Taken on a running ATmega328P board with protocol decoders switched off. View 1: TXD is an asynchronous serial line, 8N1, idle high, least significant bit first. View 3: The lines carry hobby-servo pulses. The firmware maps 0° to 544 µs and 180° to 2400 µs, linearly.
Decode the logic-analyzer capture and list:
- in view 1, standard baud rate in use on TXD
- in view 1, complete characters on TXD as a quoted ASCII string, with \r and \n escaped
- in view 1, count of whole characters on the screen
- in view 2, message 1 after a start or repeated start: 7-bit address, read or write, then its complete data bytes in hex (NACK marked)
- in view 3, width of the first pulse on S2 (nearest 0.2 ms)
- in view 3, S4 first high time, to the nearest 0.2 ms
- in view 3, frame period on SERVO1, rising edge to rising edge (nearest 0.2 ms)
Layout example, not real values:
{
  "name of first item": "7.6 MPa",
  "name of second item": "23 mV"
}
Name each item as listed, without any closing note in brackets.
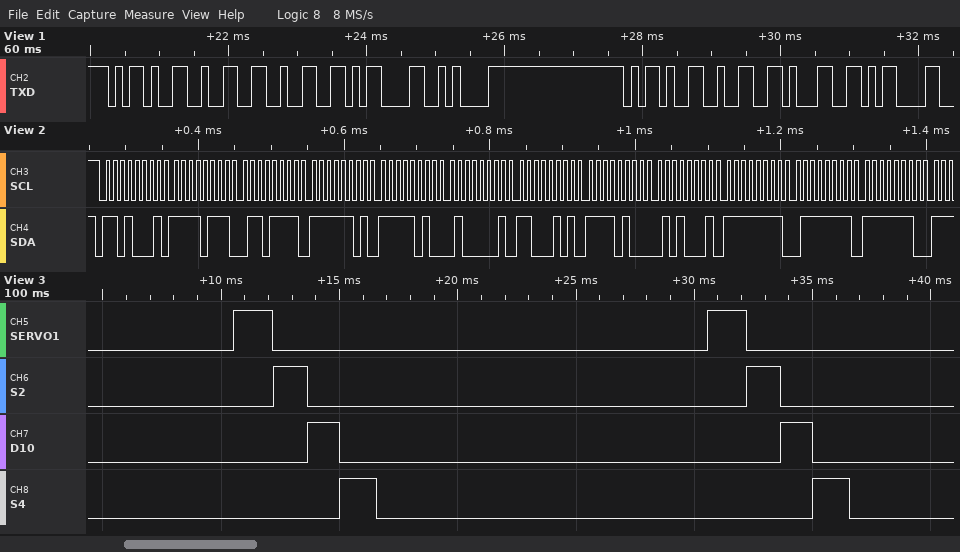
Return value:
{
  "in view 1, standard baud rate in use on TXD": "9600 baud",
  "in view 1, complete characters on TXD as a quoted ASCII string, with \\r and \\n escaped": "\"-22\\r\\n-21\\r\"",
  "in view 1, count of whole characters on the screen": "9",
  "in view 2, message 1 after a start or repeated start: 7-bit address, read or write, then its complete data bytes in hex": "0x68 read: F7 6F FD FA 41 C5 F4 51 FF 7F FE",
  "in view 3, width of the first pulse on S2": "1.4 ms",
  "in view 3, S4 first high time, to the nearest 0.2 ms": "1.6 ms",
  "in view 3, frame period on SERVO1, rising edge to rising edge": "20.0 ms"
}
